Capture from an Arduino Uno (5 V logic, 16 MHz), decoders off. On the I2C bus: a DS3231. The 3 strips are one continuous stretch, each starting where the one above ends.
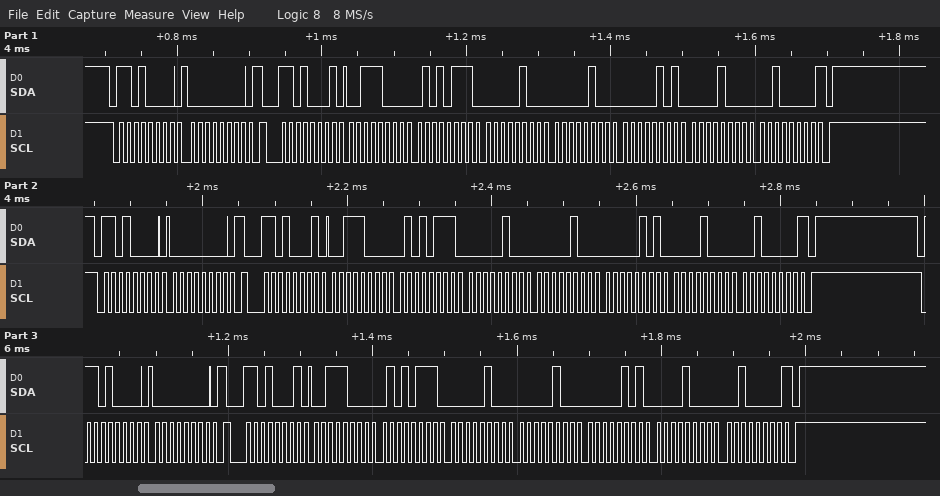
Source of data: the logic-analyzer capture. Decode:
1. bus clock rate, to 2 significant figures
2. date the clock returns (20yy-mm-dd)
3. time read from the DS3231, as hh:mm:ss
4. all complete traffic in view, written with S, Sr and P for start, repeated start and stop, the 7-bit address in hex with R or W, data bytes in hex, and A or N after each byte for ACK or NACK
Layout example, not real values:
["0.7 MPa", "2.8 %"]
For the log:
["100 kHz", "2020-08-05", "04:57:38", "S 68W A 00 A Sr 68R A 38 A 57 A 04 A 04 A 05 A 08 A 20 N P S 68W A 00 A Sr 68R A 38 A 57 A 04 A 04 A 05 A 08 A 20 N P S 68W A 00 A Sr 68R A 38 A 57 A 04 A 04 A 05 A 08 A 20 N P"]
